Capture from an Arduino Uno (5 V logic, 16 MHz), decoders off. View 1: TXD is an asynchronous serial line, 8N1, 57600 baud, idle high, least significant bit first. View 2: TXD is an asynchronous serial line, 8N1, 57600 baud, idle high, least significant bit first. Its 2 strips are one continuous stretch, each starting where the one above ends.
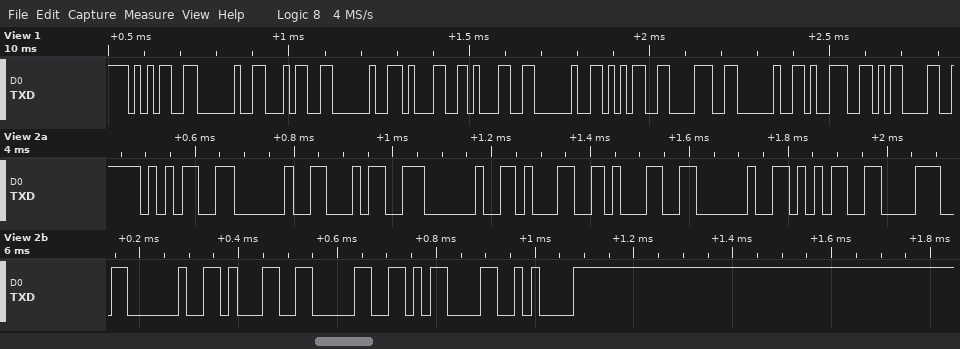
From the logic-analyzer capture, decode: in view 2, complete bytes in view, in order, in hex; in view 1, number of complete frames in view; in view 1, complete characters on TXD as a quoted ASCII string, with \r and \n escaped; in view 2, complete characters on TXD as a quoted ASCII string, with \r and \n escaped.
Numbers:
0x35 0x20 0x34 0x20 0x31 0x31 0x20 0x35 0x38 0x20 0x31 0x30 0x0D 0x0A
12
"5 4 11 58 9\r"
"5 4 11 58 10\r\n"
